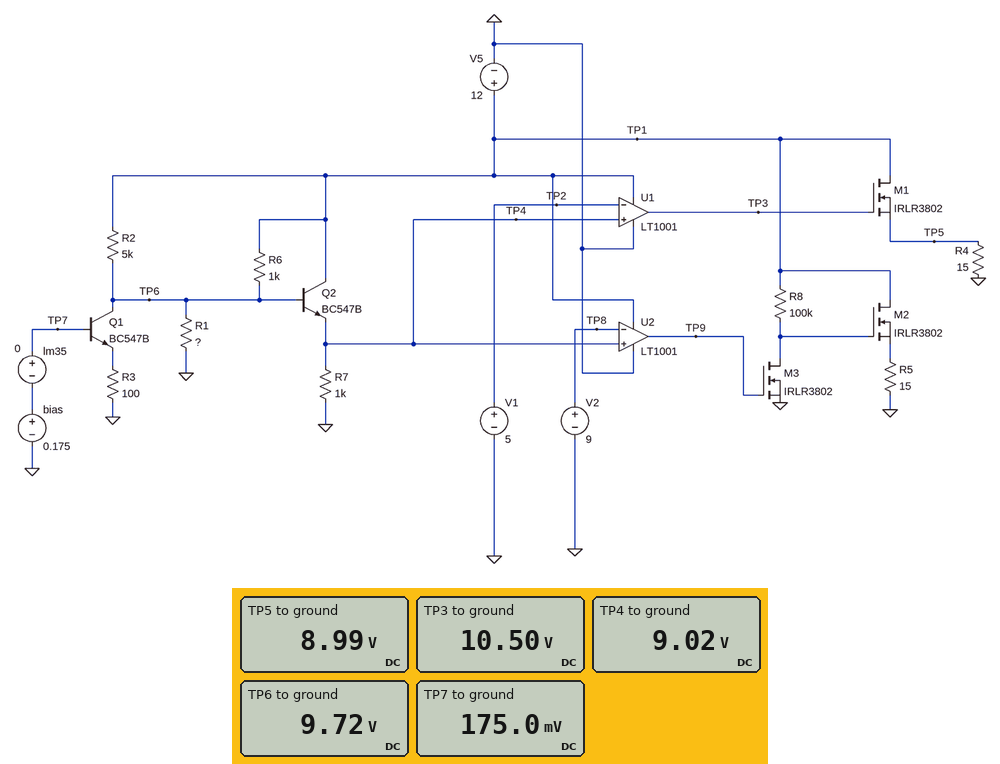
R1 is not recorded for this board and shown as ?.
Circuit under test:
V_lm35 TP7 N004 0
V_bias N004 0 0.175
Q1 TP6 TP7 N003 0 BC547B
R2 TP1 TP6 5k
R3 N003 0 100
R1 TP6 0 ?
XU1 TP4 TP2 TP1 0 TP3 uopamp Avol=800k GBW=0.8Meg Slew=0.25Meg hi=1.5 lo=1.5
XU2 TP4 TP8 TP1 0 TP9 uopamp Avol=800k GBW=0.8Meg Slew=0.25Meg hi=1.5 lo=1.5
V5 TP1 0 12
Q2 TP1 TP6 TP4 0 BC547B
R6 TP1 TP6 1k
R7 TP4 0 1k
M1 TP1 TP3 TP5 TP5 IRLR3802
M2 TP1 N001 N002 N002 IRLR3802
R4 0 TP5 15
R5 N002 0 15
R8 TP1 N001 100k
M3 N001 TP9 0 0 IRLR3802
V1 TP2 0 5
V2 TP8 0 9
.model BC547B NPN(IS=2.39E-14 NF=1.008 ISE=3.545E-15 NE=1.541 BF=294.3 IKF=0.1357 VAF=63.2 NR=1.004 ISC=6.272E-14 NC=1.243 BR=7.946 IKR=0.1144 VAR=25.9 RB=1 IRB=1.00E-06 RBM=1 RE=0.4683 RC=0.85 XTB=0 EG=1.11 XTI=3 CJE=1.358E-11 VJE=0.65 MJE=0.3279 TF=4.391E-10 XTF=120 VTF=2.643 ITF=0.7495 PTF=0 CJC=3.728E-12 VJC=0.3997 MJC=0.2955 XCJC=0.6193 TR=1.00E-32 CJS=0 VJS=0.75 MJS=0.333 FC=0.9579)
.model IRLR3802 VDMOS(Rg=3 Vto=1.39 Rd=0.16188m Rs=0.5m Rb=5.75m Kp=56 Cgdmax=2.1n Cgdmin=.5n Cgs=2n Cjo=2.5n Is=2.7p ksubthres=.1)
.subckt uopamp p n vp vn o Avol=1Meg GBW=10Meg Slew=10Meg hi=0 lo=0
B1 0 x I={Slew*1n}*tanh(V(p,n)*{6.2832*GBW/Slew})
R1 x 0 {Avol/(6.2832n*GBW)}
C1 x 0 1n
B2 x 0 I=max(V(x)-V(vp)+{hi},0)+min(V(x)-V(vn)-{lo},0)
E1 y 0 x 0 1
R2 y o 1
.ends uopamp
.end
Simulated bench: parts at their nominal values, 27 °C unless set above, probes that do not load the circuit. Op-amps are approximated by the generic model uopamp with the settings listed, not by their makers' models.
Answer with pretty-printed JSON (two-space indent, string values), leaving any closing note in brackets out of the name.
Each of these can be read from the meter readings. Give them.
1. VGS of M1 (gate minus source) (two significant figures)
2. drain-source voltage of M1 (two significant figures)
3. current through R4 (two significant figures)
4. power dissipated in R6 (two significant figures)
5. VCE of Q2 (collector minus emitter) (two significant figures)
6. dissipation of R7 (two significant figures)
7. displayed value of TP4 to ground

{
  "VGS of M1 (gate minus source)": "1.5 V",
  "drain-source voltage of M1": "3.0 V",
  "current through R4": "600 mA",
  "power dissipated in R6": "5.2 mW",
  "VCE of Q2 (collector minus emitter)": "3.0 V",
  "dissipation of R7": "81 mW",
  "displayed value of TP4 to ground": "9.02 V"
}
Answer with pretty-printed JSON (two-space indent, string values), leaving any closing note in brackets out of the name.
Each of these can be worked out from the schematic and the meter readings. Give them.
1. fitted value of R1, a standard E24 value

{
  "fitted value of R1, a standard E24 value": "3.6 kΩ"
}
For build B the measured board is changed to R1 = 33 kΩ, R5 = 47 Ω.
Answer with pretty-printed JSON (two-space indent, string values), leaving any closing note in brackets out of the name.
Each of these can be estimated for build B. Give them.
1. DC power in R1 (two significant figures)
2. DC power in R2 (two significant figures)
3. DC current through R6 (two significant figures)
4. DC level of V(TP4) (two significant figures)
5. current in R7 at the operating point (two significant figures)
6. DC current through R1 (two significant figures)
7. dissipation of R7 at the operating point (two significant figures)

{
  "DC power in R1": "4.1 mW",
  "DC power in R2": "22 µW",
  "DC current through R6": "330 µA",
  "DC level of V(TP4)": "11 V",
  "current in R7 at the operating point": "11 mA",
  "DC current through R1": "350 µA",
  "dissipation of R7 at the operating point": "120 mW"
}
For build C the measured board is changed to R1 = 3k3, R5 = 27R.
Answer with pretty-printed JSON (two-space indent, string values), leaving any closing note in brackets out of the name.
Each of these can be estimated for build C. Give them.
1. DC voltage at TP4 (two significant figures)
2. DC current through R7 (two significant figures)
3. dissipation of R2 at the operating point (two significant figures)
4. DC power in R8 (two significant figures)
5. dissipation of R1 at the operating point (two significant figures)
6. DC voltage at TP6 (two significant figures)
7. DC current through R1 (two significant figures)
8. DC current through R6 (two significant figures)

{
  "DC voltage at TP4": "8.9 V",
  "DC current through R7": "8.9 mA",
  "dissipation of R2 at the operating point": "1.2 mW",
  "DC power in R8": "1.4 mW",
  "dissipation of R1 at the operating point": "28 mW",
  "DC voltage at TP6": "9.6 V",
  "DC current through R1": "2.9 mA",
  "DC current through R6": "2.4 mA"
}
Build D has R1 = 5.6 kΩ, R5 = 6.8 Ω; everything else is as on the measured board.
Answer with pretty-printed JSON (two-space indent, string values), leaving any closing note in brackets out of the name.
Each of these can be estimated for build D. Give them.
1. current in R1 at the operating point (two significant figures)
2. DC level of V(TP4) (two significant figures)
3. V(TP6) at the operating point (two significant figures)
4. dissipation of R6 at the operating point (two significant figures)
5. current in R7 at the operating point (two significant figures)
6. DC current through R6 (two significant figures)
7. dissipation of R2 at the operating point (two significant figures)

{
  "current in R1 at the operating point": "1.9 mA",
  "DC level of V(TP4)": "9.7 V",
  "V(TP6) at the operating point": "10 V",
  "dissipation of R6 at the operating point": "2.5 mW",
  "current in R7 at the operating point": "9.7 mA",
  "DC current through R6": "1.6 mA",
  "dissipation of R2 at the operating point": "500 µW"
}
